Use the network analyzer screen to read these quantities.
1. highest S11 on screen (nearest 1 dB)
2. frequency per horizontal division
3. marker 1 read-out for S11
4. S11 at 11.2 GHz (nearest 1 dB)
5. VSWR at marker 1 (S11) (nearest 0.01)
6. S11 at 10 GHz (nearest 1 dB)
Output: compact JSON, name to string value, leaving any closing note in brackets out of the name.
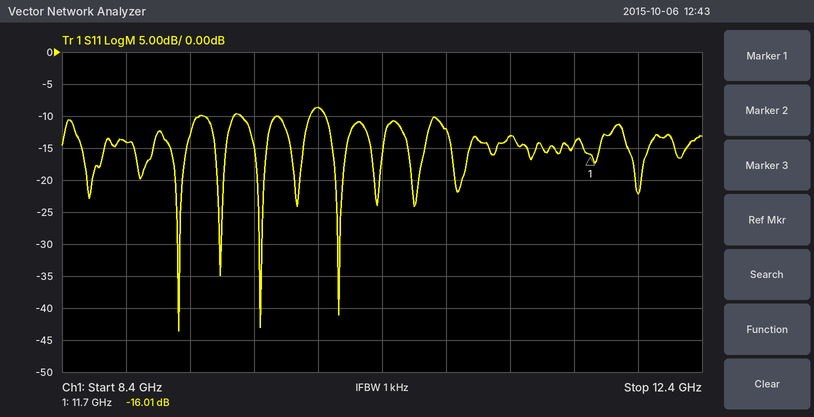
{"highest S11 on screen": "-9 dB", "frequency per horizontal division": "400 MHz", "marker 1 read-out for S11": "-16.01 dB", "S11 at 11.2 GHz": "-13 dB", "VSWR at marker 1 (S11)": "1.38", "S11 at 10 GHz": "-9 dB"}
